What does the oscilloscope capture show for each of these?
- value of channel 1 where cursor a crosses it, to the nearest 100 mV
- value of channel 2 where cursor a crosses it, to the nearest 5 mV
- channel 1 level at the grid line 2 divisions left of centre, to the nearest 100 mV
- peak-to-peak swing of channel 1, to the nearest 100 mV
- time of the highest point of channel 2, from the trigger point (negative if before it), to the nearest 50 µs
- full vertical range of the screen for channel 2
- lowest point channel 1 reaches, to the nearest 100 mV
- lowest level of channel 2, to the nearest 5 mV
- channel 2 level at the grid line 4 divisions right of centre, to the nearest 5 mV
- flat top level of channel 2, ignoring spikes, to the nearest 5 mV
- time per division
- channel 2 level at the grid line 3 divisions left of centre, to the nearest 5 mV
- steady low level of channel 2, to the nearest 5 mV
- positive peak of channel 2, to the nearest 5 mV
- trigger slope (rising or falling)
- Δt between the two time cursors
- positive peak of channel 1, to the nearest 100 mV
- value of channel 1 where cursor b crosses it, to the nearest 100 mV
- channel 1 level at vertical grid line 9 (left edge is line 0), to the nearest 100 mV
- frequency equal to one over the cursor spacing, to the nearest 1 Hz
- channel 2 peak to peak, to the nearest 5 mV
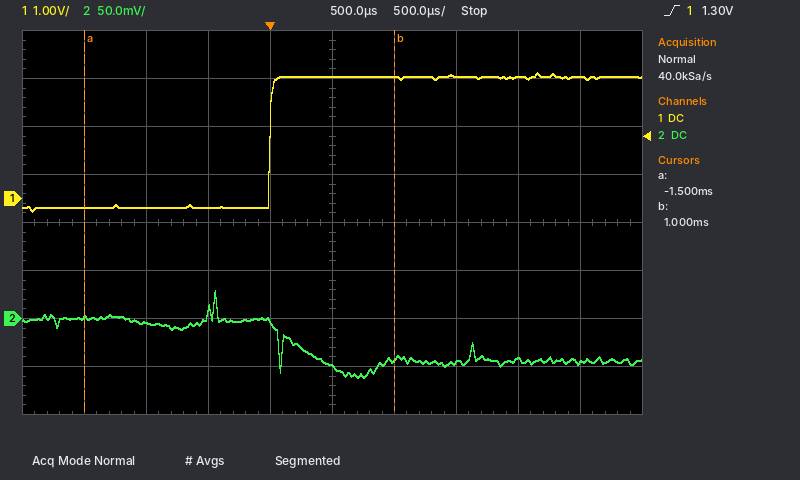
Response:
-200 mV
0 mV
-200 mV
2.9 V
-450 µs
400 mV
-300 mV
-60 mV
-45 mV
0 mV
500 µs
-5 mV
-45 mV
30 mV
rising
2.50 ms
2.6 V
2.5 V
2.5 V
400 Hz
90 mV
